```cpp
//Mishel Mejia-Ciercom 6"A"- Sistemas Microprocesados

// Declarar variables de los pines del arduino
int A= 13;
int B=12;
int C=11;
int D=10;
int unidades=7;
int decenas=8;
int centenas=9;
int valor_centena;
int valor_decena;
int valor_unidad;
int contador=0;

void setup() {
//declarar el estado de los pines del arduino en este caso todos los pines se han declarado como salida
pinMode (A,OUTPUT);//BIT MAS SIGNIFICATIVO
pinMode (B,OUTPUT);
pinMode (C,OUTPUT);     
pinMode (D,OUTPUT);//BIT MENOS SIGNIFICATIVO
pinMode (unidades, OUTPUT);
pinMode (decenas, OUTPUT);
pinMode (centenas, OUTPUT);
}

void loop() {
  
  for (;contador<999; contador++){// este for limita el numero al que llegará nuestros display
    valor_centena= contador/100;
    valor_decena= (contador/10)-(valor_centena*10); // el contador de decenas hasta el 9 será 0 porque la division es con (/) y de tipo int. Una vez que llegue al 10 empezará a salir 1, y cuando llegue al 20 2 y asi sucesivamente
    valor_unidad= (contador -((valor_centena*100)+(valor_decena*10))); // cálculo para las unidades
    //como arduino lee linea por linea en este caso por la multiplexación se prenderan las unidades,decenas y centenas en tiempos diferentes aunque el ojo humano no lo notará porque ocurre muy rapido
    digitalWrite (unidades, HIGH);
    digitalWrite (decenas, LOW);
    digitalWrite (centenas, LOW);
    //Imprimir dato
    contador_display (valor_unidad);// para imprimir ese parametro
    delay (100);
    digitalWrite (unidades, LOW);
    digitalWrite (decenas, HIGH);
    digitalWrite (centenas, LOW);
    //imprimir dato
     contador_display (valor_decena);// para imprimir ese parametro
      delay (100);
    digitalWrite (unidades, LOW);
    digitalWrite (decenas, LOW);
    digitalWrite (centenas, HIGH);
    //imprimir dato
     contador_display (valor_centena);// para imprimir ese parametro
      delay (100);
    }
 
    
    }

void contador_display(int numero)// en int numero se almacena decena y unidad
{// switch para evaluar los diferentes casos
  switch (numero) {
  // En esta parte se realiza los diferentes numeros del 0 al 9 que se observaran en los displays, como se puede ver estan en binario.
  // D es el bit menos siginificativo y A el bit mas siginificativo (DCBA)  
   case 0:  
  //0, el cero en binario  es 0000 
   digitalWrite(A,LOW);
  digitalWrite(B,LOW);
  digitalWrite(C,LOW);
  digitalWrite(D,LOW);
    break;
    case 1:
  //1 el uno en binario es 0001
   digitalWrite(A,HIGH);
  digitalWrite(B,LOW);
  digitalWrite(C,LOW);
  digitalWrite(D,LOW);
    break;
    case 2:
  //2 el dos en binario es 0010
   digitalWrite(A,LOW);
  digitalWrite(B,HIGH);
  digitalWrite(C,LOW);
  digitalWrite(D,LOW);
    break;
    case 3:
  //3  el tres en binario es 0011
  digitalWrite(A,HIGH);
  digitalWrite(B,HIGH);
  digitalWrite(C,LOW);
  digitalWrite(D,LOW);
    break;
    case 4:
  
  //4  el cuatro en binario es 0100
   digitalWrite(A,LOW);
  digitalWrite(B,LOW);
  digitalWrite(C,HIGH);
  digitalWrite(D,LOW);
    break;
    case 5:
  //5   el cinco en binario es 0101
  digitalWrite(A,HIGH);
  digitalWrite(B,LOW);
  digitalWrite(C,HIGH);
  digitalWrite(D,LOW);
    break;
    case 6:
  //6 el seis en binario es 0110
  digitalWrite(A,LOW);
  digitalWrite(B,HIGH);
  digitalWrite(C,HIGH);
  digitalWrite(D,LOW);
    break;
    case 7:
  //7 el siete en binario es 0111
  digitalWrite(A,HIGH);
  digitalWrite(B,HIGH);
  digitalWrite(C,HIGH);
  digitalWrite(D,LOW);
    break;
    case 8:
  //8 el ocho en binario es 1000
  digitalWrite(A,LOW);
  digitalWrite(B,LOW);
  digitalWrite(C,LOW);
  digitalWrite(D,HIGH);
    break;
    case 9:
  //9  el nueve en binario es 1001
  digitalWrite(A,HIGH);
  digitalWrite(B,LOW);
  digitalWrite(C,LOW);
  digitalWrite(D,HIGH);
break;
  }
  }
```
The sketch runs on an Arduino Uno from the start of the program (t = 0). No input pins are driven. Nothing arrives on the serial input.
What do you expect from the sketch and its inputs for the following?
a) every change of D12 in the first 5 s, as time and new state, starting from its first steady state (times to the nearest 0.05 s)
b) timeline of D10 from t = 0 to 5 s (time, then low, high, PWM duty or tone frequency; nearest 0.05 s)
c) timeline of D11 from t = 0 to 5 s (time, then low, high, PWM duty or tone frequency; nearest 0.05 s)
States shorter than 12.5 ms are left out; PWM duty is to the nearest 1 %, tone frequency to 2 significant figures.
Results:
0 s low; 0.6 s high; 0.7 s low; 0.9 s high; 1 s low; 1.8 s high; 1.9 s low; 2.1 s high; 2.2 s low; 3.6 s high; 3.7 s low; 3.9 s high; 4 s low; 4.8 s high; 4.9 s low
0 s low; 2.4 s high; 2.5 s low; 2.7 s high; 2.8 s low
0 s low; 1.2 s high; 1.3 s low; 1.5 s high; 1.6 s low; 1.8 s high; 1.9 s low; 2.1 s high; 2.2 s low; 4.2 s high; 4.3 s low; 4.5 s high; 4.6 s low; 4.8 s high; 4.9 s low
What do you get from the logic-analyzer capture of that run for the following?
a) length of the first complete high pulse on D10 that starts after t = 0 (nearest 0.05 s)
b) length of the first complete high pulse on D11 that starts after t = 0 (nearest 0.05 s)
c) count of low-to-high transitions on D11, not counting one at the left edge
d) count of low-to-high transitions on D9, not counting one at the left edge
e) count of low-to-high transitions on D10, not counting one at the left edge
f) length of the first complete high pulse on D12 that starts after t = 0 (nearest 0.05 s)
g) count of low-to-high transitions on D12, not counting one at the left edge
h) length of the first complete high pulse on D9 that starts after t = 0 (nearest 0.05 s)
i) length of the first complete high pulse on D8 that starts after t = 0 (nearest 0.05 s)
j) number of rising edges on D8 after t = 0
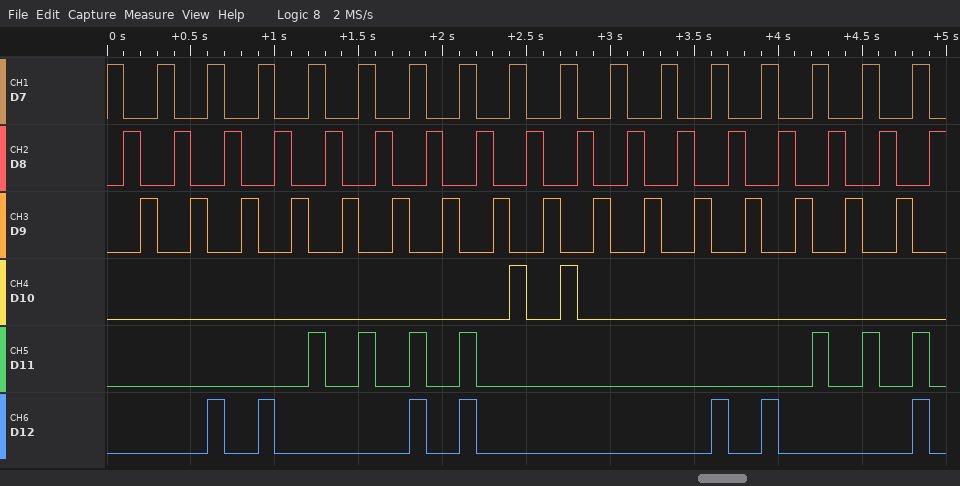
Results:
0.10 s
0.10 s
7
16
2
0.10 s
7
0.10 s
0.10 s
17
